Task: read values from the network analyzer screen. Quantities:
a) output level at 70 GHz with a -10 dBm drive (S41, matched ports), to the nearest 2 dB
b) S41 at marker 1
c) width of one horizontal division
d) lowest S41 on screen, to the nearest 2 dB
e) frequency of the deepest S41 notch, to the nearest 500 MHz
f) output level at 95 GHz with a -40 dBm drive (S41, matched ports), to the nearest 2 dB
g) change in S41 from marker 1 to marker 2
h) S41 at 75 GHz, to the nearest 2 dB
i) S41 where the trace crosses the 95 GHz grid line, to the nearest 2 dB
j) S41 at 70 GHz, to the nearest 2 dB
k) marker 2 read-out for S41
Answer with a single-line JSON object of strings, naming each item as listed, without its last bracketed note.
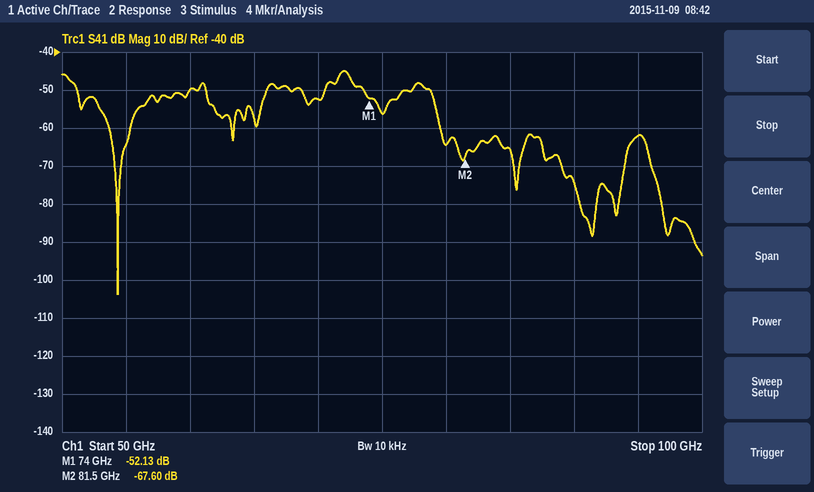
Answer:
{"output level at 70 GHz with a -10 dBm drive (S41, matched ports), to the nearest 2 dB": "-62 dBm", "S41 at marker 1": "-52.13 dB", "width of one horizontal division": "5 GHz", "lowest S41 on screen, to the nearest 2 dB": "-104 dB", "frequency of the deepest S41 notch, to the nearest 500 MHz": "54.5 GHz", "output level at 95 GHz with a -40 dBm drive (S41, matched ports), to the nearest 2 dB": "-102 dBm", "change in S41 from marker 1 to marker 2": "-15.47 dB", "S41 at 75 GHz, to the nearest 2 dB": "-56 dB", "S41 where the trace crosses the 95 GHz grid line, to the nearest 2 dB": "-62 dB", "S41 at 70 GHz, to the nearest 2 dB": "-52 dB", "marker 2 read-out for S41": "-67.60 dB"}
